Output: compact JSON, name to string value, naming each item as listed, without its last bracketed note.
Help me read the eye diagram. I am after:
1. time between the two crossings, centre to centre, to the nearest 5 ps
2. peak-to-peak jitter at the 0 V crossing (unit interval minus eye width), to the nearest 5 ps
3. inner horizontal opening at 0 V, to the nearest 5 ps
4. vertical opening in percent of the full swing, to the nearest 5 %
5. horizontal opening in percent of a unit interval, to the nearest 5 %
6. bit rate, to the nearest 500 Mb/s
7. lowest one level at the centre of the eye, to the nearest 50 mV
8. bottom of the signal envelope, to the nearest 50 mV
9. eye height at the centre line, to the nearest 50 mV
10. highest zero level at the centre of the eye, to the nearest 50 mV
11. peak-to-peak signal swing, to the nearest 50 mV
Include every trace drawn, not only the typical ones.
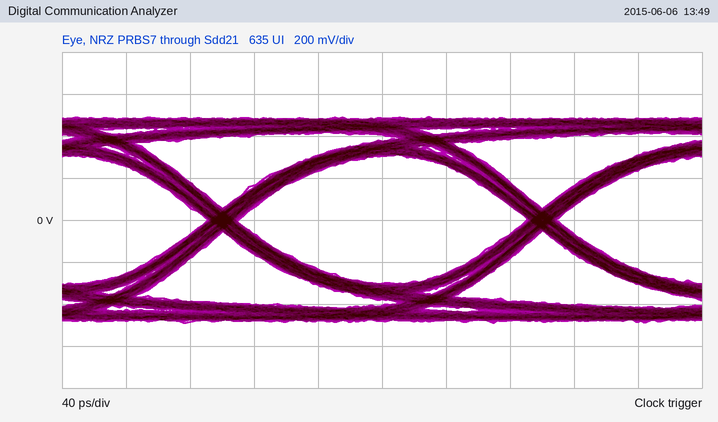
{"time between the two crossings, centre to centre, to the nearest 5 ps": "200 ps", "peak-to-peak jitter at the 0 V crossing (unit interval minus eye width), to the nearest 5 ps": "20 ps", "inner horizontal opening at 0 V, to the nearest 5 ps": "180 ps", "vertical opening in percent of the full swing, to the nearest 5 %": "60 %", "horizontal opening in percent of a unit interval, to the nearest 5 %": "90 %", "bit rate, to the nearest 500 Mb/s": "5.0 Gb/s", "lowest one level at the centre of the eye, to the nearest 50 mV": "300 mV", "bottom of the signal envelope, to the nearest 50 mV": "-500 mV", "eye height at the centre line, to the nearest 50 mV": "600 mV", "highest zero level at the centre of the eye, to the nearest 50 mV": "-300 mV", "peak-to-peak signal swing, to the nearest 50 mV": "1.00 V"}
